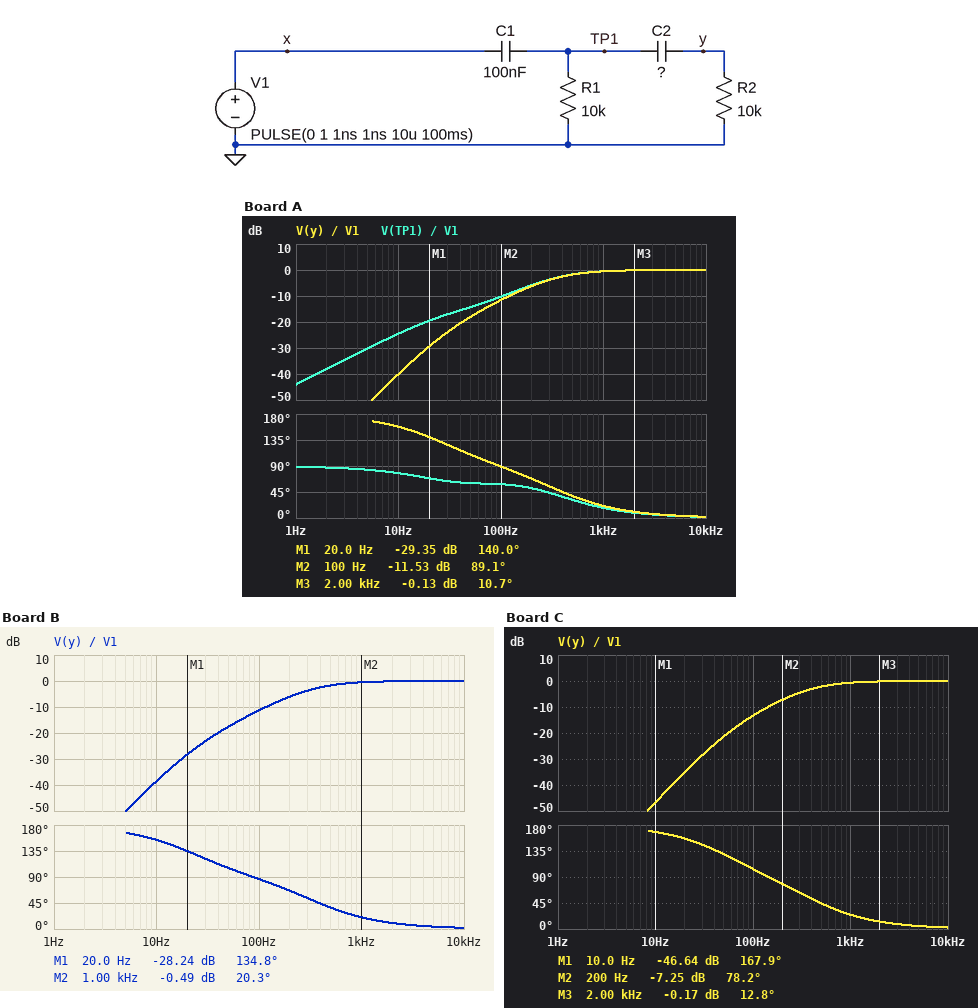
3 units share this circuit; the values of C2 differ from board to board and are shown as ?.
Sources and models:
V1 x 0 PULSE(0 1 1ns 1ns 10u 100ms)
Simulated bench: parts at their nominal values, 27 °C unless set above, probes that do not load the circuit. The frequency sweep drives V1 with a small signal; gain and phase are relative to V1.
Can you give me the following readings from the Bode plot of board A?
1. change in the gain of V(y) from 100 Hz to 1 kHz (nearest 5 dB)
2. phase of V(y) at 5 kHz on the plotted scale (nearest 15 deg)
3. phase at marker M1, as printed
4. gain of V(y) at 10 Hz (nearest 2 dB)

10 dB
0 deg
140.0 deg
-40 dB
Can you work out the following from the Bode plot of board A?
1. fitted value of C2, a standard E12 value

270 nF
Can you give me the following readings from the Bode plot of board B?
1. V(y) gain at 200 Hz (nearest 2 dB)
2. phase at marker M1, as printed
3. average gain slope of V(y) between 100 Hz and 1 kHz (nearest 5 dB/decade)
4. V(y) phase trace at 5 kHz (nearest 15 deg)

-6 dB
134.8 deg
10 dB/decade
0 deg
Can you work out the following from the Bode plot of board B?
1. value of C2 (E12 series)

330 nF
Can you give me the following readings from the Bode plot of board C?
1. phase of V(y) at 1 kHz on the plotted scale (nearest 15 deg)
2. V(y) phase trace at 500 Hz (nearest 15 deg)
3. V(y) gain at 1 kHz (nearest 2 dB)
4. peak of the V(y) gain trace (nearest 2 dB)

30 deg
45 deg
0 dB
0 dB
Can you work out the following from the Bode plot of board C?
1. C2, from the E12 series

120 nF
